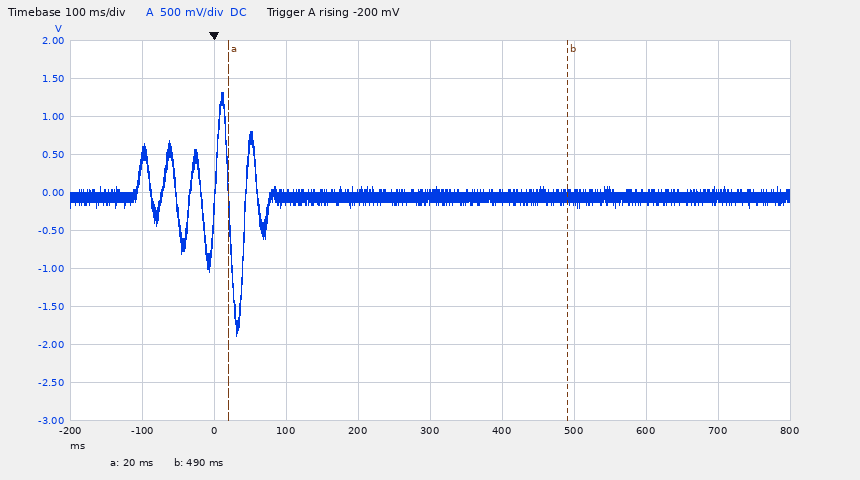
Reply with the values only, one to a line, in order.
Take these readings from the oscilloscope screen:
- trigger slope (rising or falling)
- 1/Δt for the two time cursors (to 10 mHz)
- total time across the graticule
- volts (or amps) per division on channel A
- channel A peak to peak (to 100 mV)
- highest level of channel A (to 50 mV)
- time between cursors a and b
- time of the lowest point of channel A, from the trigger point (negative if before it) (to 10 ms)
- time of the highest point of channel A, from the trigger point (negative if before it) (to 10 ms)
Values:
rising
2.13 Hz
1 s
500 mV
3.20 V
1.30 V
470 ms
+30 ms
+10 ms
